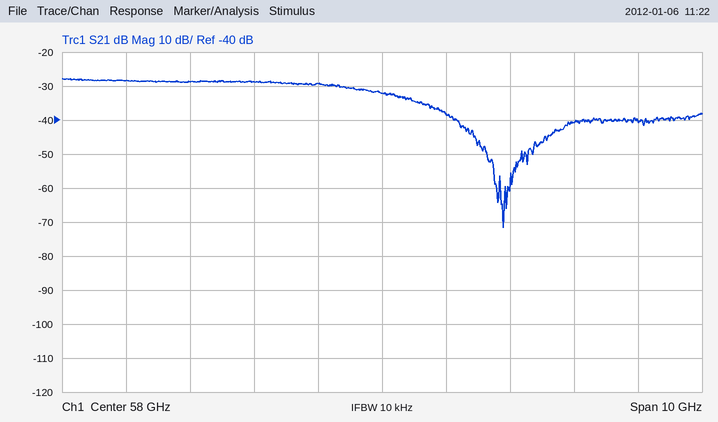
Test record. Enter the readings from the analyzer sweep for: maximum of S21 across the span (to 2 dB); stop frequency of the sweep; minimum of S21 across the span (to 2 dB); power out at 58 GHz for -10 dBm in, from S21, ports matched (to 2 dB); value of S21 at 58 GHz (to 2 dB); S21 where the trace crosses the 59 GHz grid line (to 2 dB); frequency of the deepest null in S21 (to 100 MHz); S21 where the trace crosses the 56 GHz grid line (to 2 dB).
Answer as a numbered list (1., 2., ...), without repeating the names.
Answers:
1. -28 dB
2. 63 GHz
3. -72 dB
4. -42 dBm
5. -32 dB
6. -38 dB
7. 59.9 GHz
8. -28 dB
